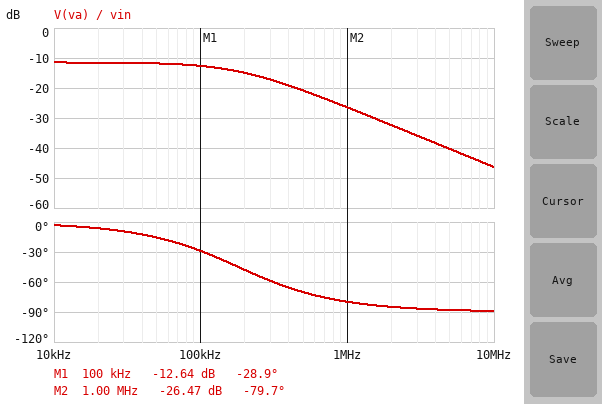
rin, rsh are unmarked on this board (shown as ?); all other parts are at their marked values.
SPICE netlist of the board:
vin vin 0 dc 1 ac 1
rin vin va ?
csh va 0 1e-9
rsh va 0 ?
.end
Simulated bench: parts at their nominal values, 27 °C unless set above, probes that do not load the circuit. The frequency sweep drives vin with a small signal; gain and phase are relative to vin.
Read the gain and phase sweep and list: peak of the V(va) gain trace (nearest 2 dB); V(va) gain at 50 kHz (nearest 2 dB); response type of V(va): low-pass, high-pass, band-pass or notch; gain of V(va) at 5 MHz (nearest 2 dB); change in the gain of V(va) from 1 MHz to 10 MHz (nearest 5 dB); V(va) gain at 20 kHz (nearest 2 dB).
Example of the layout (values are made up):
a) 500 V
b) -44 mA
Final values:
a) -12 dB
b) -12 dB
c) low-pass
d) -40 dB
e) -20 dB
f) -12 dB
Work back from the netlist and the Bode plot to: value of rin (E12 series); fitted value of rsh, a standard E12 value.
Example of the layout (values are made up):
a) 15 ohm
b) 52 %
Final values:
a) 3.3 kΩ
b) 1.2 kΩ
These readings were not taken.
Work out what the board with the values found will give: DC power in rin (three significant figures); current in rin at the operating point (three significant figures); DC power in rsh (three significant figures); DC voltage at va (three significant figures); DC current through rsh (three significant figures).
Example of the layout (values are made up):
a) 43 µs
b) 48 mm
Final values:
a) 163 µW
b) 222 µA
c) 59.3 µW
d) 267 mV
e) 222 µA
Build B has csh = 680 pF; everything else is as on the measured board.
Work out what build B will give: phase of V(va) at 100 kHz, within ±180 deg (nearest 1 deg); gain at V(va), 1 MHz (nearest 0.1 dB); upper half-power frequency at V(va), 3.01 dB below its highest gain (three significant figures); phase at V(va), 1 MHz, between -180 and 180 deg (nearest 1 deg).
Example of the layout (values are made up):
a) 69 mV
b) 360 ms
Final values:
a) -21 deg
b) -23.3 dB
c) 266 kHz
d) -75 deg
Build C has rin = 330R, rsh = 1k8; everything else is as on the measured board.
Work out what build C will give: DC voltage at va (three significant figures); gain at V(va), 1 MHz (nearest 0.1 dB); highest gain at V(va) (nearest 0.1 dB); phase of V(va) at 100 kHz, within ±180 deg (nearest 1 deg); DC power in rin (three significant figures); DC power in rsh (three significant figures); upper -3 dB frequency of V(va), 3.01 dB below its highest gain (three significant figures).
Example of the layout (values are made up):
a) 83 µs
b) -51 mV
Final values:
a) 845 mV
b) -7.6 dB
c) -1.5 dB
d) -10 deg
e) 72.7 µW
f) 397 µW
g) 571 kHz
